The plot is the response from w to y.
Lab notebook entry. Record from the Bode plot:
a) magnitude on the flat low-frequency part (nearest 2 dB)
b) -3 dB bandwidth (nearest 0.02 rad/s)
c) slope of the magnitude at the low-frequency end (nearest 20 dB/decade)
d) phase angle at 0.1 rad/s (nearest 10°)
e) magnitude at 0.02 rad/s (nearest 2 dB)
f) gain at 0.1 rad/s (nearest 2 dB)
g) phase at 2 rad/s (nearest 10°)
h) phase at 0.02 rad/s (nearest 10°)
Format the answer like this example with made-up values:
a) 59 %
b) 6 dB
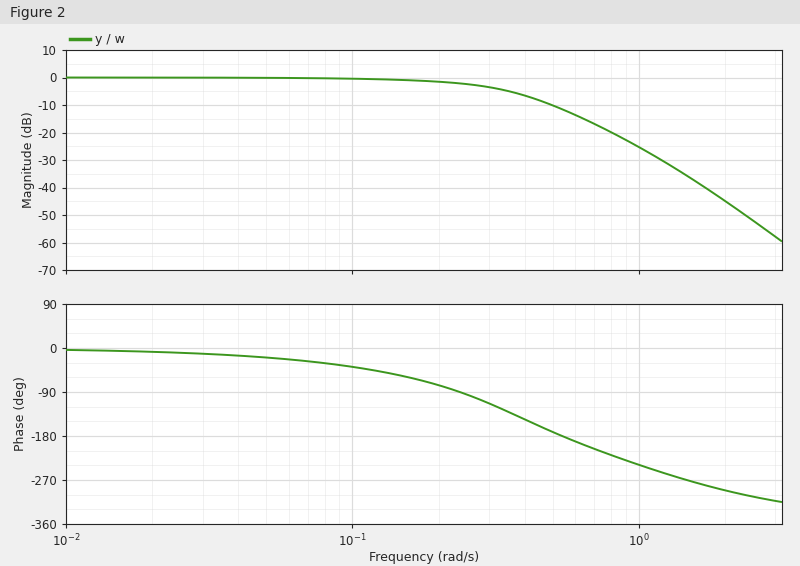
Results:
a) 0 dB
b) 0.28 rad/s
c) 0 dB/decade
d) -40°
e) 0 dB
f) 0 dB
g) -290°
h) -10°
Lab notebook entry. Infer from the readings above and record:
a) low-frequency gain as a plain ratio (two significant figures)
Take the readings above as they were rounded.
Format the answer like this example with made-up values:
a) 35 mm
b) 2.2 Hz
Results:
a) 1.0
